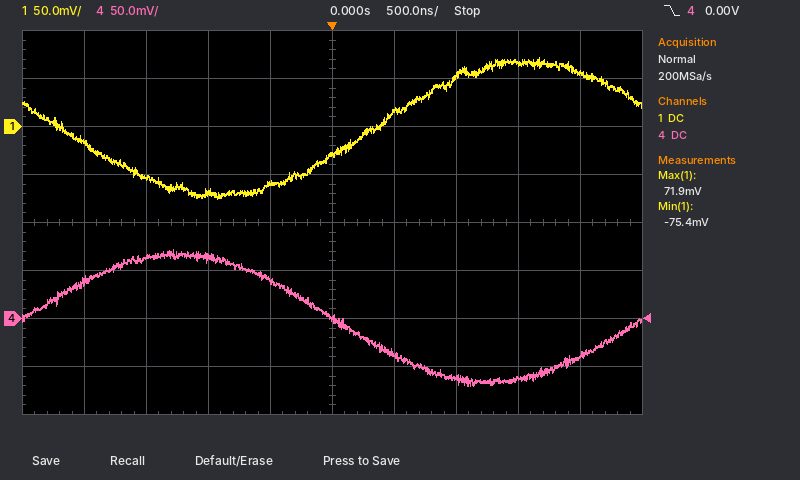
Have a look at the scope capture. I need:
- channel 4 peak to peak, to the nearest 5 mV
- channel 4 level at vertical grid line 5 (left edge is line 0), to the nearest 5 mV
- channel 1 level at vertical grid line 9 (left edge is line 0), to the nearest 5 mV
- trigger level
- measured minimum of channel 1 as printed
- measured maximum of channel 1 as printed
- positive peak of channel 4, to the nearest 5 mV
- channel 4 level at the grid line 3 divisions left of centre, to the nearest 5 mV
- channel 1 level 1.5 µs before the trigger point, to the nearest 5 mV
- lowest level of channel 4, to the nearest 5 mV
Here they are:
140 mV
0 mV
55 mV
0.00 V
-75.4 mV
71.9 mV
70 mV
65 mV
-55 mV
-70 mV
